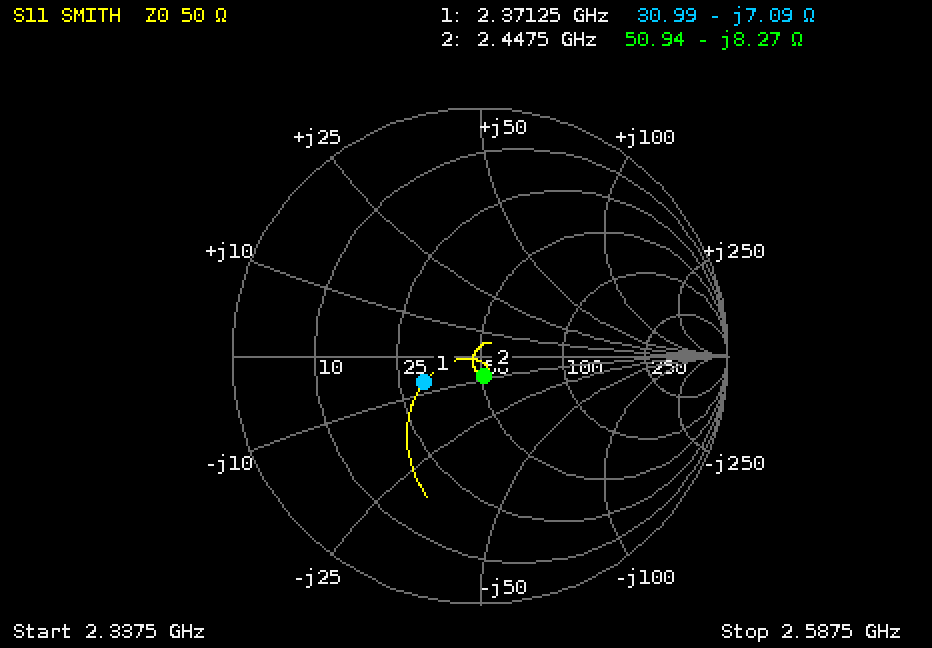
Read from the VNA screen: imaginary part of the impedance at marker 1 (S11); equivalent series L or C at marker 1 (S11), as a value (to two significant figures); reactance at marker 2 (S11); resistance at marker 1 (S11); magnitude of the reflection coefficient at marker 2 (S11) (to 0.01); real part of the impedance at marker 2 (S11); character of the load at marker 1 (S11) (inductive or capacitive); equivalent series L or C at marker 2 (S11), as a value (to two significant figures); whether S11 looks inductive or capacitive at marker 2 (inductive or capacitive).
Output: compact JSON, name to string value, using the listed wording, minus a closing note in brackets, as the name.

{"imaginary part of the impedance at marker 1": "-7.09 Ω", "equivalent series L or C at marker 1 (S11), as a value": "9.5 pF", "reactance at marker 2": "-8.27 Ω", "resistance at marker 1": "30.99 Ω", "magnitude of the reflection coefficient at marker 2 (S11)": "0.08", "real part of the impedance at marker 2": "50.94 Ω", "character of the load at marker 1 (S11)": "capacitive", "equivalent series L or C at marker 2 (S11), as a value": "7.9 pF", "whether S11 looks inductive or capacitive at marker 2": "capacitive"}
